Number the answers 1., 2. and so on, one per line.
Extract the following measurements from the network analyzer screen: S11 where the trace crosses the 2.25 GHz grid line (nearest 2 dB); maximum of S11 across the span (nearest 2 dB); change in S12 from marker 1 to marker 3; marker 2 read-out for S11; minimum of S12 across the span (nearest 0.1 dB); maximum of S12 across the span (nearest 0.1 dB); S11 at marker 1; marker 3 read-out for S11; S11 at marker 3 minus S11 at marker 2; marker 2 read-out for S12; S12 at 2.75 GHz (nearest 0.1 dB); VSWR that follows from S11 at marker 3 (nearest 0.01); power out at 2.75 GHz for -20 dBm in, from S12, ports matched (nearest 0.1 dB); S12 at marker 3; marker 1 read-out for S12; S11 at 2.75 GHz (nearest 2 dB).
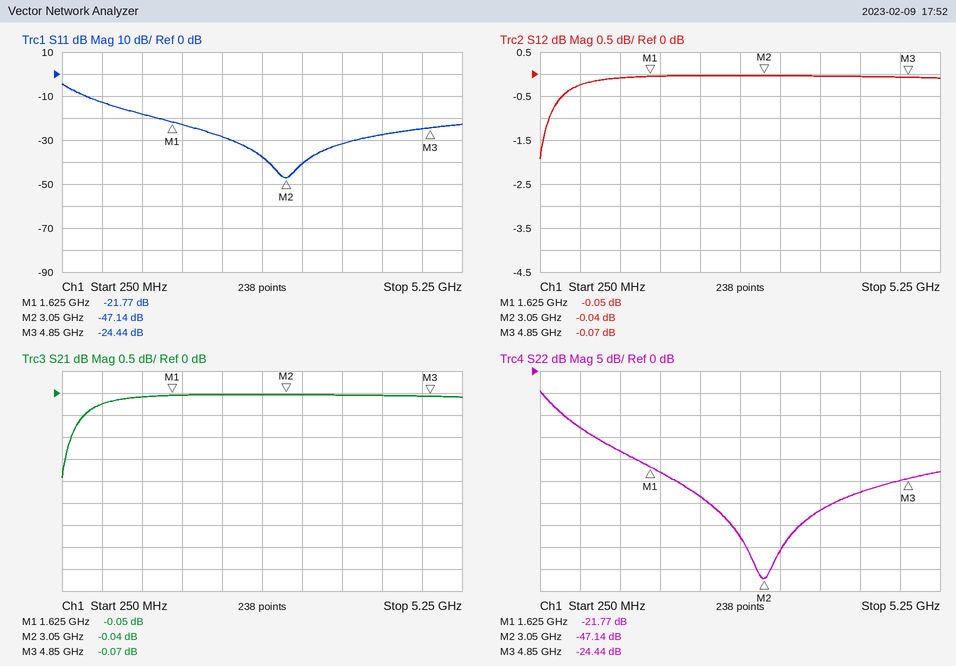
1. -28 dB
2. -4 dB
3. -0.02 dB
4. -47.14 dB
5. -1.9 dB
6. 0.0 dB
7. -21.77 dB
8. -24.44 dB
9. 22.70 dB
10. -0.04 dB
11. 0.0 dB
12. 1.13
13. -20.0 dBm
14. -0.07 dB
15. -0.05 dB
16. -38 dB
